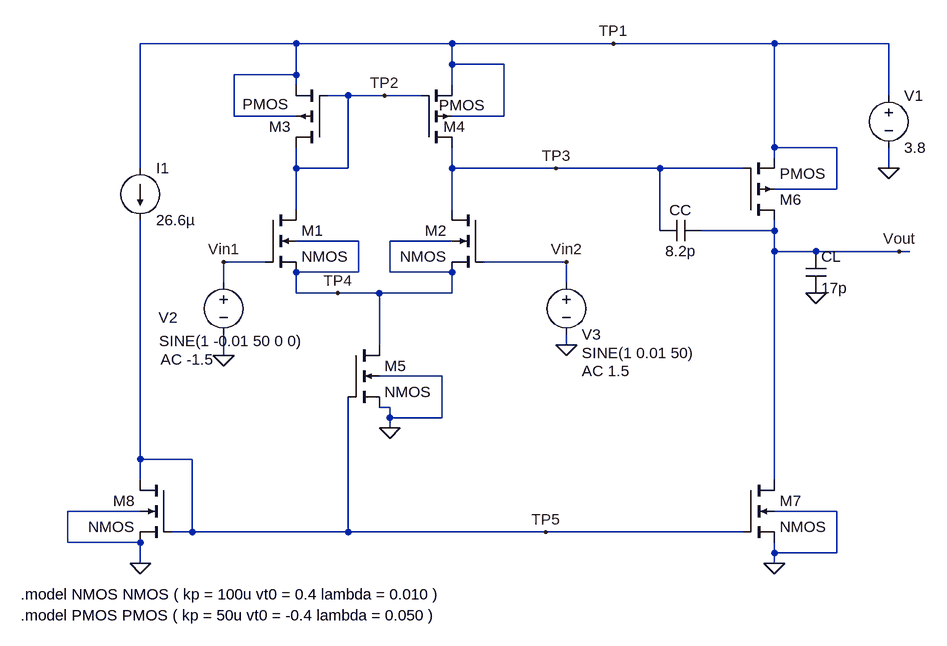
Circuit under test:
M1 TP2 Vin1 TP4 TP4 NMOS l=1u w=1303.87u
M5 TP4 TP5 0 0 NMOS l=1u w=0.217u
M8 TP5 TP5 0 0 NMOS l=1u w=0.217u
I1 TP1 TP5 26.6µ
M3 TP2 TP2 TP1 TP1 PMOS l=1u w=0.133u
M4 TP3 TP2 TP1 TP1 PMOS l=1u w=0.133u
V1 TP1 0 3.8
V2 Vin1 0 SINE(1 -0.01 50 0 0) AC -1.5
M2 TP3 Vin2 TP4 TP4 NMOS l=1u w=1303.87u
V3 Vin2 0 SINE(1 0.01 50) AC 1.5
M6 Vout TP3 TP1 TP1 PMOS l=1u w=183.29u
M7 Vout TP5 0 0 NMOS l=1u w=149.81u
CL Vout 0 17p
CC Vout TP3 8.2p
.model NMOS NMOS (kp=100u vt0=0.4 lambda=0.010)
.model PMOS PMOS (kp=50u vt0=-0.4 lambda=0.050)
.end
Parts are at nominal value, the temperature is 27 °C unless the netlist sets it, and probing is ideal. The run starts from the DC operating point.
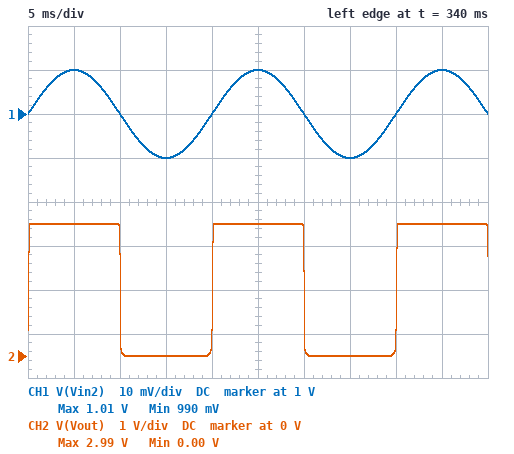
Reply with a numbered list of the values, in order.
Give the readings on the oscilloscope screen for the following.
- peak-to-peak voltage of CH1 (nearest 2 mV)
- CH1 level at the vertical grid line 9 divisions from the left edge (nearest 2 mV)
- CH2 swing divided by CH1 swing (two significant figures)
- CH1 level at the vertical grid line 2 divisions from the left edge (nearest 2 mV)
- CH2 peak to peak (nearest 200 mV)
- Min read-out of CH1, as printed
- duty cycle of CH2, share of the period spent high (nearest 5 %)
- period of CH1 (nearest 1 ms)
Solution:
1. 20 mV
2. 1.010 V
3. 150
4. 1.000 V
5. 3.0 V
6. 990 mV
7. 50 %
8. 20 ms
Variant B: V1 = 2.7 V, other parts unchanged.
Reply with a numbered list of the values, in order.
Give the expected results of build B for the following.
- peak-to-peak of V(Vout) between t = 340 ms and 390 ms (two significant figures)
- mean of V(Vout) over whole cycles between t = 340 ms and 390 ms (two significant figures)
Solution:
1. 880 mV
2. 440 mV
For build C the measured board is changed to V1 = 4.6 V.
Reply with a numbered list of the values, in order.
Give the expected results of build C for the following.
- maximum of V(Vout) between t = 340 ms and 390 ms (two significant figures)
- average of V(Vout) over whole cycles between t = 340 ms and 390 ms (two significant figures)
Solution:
1. 4.0 V
2. 2.0 V
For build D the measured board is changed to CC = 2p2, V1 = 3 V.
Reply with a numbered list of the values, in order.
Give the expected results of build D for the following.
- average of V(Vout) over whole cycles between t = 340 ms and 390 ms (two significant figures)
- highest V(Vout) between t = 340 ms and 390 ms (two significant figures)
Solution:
1. 780 mV
2. 1.6 V
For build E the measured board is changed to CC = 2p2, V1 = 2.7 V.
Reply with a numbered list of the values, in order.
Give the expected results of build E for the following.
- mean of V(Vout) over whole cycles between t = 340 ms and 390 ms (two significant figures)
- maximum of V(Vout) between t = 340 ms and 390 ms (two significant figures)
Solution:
1. 440 mV
2. 880 mV
